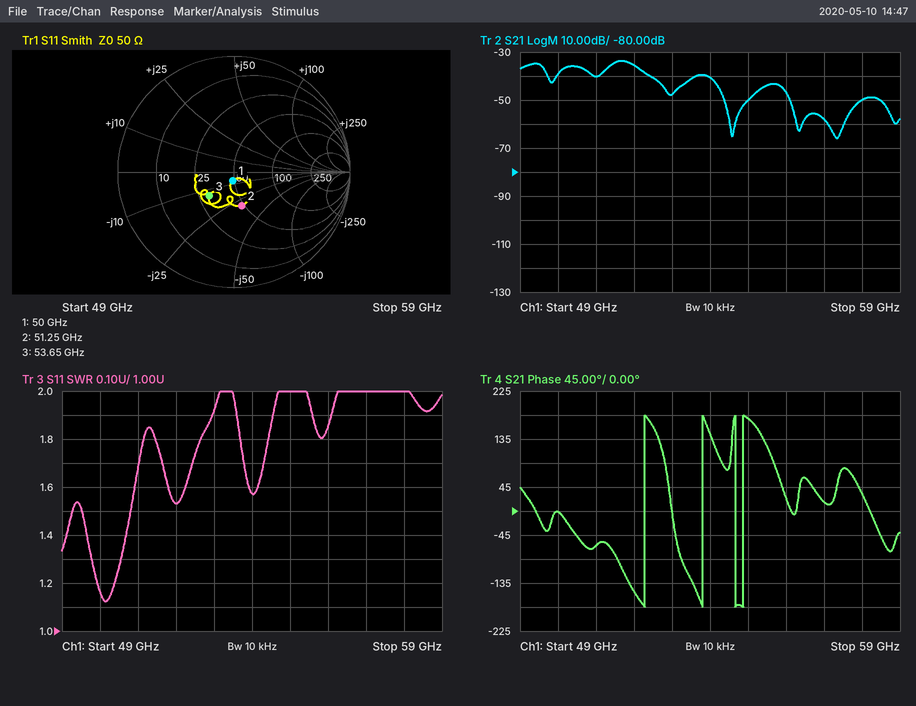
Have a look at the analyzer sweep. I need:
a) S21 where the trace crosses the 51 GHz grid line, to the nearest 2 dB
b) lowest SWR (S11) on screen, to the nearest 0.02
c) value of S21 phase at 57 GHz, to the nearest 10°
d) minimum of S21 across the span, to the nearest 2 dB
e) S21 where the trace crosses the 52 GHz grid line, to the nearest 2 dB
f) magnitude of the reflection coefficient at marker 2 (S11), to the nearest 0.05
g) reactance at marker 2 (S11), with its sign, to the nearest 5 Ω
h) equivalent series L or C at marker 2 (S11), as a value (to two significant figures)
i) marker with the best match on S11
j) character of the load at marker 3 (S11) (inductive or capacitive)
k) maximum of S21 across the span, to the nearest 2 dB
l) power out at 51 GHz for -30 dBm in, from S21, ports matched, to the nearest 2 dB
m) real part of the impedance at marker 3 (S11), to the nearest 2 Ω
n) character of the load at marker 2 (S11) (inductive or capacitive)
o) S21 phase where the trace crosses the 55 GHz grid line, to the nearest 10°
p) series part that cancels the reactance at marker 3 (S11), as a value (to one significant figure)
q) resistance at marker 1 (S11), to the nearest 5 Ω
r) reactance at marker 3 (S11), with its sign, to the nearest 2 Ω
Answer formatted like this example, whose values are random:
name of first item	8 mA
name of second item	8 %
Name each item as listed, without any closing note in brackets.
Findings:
S21 where the trace crosses the 51 GHz grid line, to the nearest 2 dB	-40 dB
lowest SWR (S11) on screen, to the nearest 0.02	1.12
value of S21 phase at 57 GHz, to the nearest 10°	20°
minimum of S21 across the span, to the nearest 2 dB	-66 dB
S21 where the trace crosses the 52 GHz grid line, to the nearest 2 dB	-36 dB
magnitude of the reflection coefficient at marker 2 (S11), to the nearest 0.05	0.30
reactance at marker 2 (S11), with its sign, to the nearest 5 Ω	-30 Ω
equivalent series L or C at marker 2 (S11), as a value	100 fF
marker with the best match on S11	marker 1
character of the load at marker 3 (S11)	capacitive
maximum of S21 across the span, to the nearest 2 dB	-34 dB
power out at 51 GHz for -30 dBm in, from S21, ports matched, to the nearest 2 dB	-70 dBm
real part of the impedance at marker 3 (S11), to the nearest 2 Ω	30 Ω
character of the load at marker 2 (S11)	capacitive
S21 phase where the trace crosses the 55 GHz grid line, to the nearest 10°	170°
series part that cancels the reactance at marker 3 (S11), as a value	40 pH
resistance at marker 1 (S11), to the nearest 5 Ω	50 Ω
reactance at marker 3 (S11), with its sign, to the nearest 2 Ω	-14 Ω
